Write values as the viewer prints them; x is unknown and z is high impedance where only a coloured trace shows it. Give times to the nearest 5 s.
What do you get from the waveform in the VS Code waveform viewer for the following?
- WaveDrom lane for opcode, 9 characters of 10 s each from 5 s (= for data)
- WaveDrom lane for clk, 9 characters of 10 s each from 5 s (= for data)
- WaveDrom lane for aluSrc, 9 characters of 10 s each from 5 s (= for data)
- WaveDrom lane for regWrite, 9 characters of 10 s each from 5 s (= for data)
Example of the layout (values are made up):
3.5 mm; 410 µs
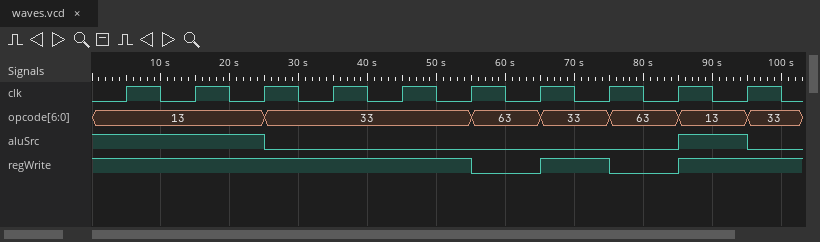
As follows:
{name: 'opcode', wave: '=.=..====', data: '13 33 63 33 63 13'}; {name: 'clk', wave: 'p........'}; {name: 'aluSrc', wave: '1.0.....1'}; {name: 'regWrite', wave: '1....0101'}
